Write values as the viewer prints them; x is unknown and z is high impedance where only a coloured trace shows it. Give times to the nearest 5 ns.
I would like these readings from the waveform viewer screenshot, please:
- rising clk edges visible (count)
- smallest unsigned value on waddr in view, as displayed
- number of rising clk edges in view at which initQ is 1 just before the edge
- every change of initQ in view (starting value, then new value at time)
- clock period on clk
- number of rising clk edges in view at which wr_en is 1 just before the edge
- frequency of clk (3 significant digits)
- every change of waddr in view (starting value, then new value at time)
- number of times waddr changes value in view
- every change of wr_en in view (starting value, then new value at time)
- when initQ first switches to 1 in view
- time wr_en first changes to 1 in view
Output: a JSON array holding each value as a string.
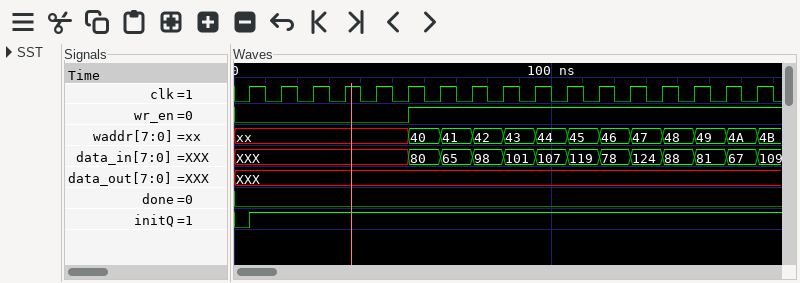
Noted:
["17", "40", "16", "0, 1 at 5 ns", "10 ns", "11", "100 MHz", "xx, 40 at 55 ns, 41 at 65 ns, 42 at 75 ns, 43 at 85 ns, 44 at 95 ns, 45 at 105 ns, 46 at 115 ns, 47 at 125 ns, 48 at 135 ns, 49 at 145 ns, 4A at 155 ns, 4B at 165 ns", "12", "0, 1 at 55 ns", "5 ns", "55 ns"]
